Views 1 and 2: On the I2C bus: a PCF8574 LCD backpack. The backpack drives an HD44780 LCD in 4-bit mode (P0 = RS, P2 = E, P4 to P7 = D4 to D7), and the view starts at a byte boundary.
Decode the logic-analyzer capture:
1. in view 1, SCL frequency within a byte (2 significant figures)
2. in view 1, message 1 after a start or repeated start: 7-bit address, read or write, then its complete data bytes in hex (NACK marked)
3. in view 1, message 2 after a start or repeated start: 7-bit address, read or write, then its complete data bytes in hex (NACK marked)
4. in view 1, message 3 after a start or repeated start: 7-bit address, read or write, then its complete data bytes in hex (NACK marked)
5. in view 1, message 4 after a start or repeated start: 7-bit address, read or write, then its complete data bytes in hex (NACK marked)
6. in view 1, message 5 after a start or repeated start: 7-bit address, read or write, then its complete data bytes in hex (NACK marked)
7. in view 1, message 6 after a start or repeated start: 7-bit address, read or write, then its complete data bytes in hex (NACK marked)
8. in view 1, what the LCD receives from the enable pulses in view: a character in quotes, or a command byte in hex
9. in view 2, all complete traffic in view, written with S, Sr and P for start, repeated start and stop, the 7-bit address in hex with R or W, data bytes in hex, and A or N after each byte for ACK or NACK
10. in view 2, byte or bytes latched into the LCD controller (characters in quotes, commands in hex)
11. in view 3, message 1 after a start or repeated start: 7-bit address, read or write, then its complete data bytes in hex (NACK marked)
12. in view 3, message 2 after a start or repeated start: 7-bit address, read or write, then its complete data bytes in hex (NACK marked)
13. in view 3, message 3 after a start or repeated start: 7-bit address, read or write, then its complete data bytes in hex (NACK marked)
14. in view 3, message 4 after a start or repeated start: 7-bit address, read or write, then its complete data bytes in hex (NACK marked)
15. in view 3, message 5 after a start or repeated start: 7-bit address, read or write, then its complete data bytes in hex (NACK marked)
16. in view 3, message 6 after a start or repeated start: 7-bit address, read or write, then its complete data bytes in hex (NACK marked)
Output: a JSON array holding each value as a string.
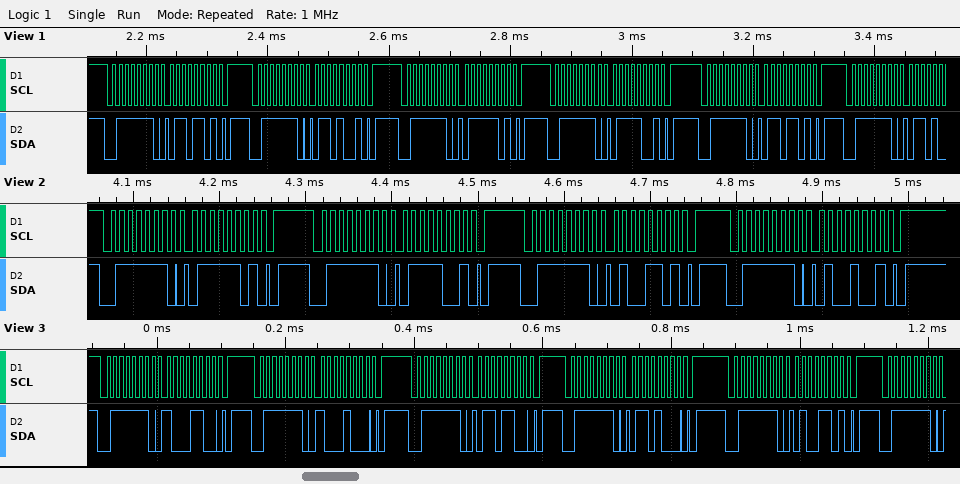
["100 kHz", "0x3F write: 6D", "0x3F write: 69", "0x3F write: 7D", "0x3F write: 79", "0x3F write: 6D", "0x3F write", "'g'", "S 3FW A 7D A P S 3FW A 79 A P S 3FW A 4D A P S 3FW A 49 A P", "'t'", "0x3F write: 8C", "0x3F write: 88", "0x3F write: 6C", "0x3F write: 68", "0x3F write: 4D", "0x3F write"]
